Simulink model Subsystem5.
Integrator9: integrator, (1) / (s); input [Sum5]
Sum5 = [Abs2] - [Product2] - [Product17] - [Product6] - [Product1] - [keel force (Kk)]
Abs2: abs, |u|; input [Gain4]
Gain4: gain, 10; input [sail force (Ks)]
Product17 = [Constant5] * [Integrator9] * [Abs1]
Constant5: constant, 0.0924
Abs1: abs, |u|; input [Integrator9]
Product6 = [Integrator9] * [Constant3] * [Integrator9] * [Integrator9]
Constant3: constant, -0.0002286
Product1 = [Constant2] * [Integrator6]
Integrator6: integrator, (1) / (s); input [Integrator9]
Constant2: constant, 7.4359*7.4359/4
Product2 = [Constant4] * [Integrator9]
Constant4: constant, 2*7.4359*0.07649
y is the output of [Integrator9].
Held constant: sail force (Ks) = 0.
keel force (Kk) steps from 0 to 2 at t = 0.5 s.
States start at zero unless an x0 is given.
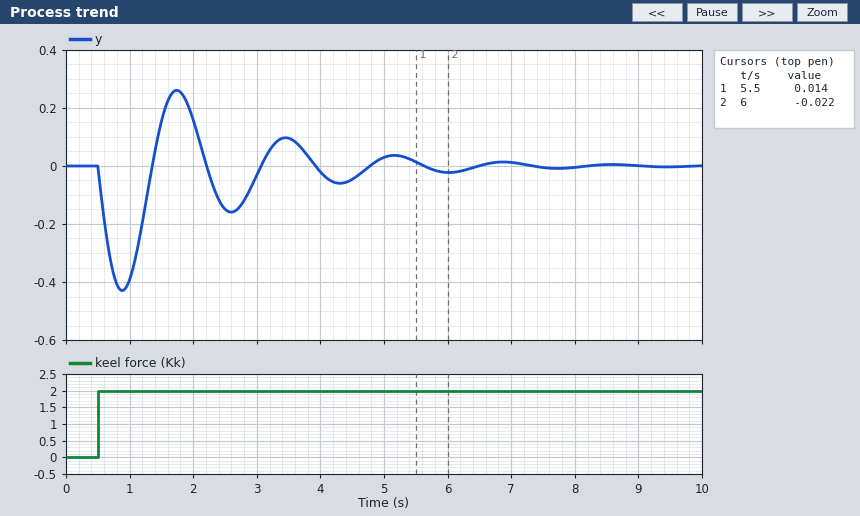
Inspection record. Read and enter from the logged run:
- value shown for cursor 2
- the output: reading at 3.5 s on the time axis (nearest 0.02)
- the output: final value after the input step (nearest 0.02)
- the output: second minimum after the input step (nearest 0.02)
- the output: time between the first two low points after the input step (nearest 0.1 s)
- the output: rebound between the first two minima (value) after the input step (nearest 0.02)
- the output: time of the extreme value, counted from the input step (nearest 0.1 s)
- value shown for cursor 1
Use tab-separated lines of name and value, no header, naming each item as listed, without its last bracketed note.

value shown for cursor 2	-0.022
the output: reading at 3.5 s on the time axis	0.10
the output: final value after the input step	0.00
the output: second minimum after the input step	-0.16
the output: time between the first two low points after the input step	1.7 s
the output: rebound between the first two minima (value) after the input step	0.26
the output: time of the extreme value, counted from the input step	0.4 s
value shown for cursor 1	0.014
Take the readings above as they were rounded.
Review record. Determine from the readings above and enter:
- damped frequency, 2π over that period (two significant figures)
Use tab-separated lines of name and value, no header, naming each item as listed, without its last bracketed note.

damped frequency, 2π over that period	3.7 rad/s
